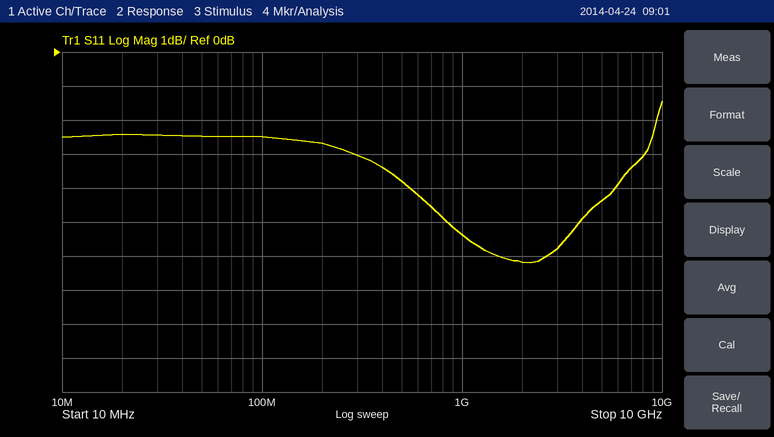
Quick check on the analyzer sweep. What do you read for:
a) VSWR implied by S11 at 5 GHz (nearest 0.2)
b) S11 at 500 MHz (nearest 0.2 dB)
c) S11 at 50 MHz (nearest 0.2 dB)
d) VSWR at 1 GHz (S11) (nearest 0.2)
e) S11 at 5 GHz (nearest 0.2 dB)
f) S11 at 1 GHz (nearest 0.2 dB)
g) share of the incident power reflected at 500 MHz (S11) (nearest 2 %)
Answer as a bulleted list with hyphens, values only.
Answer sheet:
- 4.0
- -3.8 dB
- -2.4 dB
- 3.4
- -4.4 dB
- -5.4 dB
- 42 %
